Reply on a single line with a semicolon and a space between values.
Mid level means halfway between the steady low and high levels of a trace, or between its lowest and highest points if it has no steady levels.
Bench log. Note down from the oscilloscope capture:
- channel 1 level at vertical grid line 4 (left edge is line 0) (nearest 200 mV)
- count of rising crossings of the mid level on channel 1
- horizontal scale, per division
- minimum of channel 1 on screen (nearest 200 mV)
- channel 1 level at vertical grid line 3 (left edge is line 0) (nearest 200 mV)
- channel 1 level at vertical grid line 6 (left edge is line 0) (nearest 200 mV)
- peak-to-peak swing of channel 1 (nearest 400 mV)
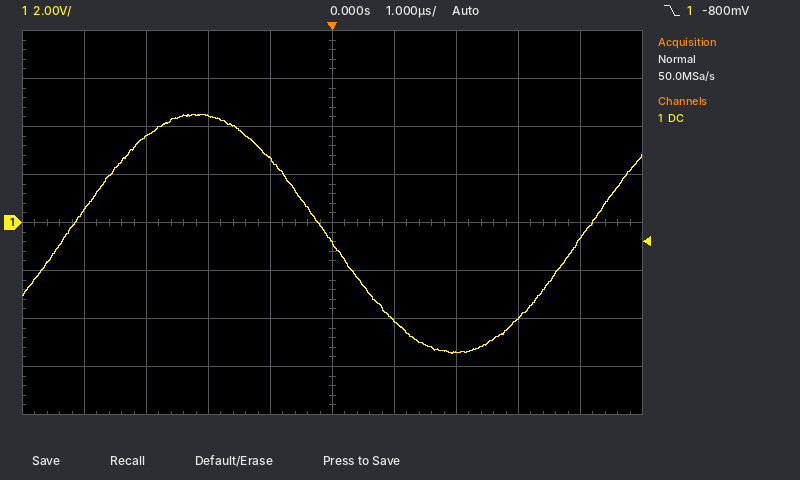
2.6 V; 2; 1 µs; -5.4 V; 4.4 V; -4.0 V; 10.0 V
